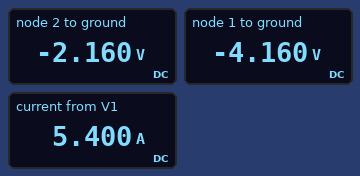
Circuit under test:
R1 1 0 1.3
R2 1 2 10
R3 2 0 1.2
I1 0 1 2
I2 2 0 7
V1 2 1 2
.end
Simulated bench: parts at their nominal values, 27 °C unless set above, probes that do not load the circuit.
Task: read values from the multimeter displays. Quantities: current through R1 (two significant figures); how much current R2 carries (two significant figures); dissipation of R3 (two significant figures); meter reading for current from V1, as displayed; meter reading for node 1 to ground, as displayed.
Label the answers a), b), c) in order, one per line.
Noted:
a) 3.2 A
b) 200 mA
c) 3.9 W
d) 5.400 A
e) -4.160 V
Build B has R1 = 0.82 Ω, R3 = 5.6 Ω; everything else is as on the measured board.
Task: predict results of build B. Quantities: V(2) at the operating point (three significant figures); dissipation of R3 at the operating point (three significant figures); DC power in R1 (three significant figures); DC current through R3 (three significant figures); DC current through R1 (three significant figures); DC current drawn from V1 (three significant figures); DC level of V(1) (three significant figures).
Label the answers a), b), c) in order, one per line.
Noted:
a) -1.83 V
b) 599 mW
c) 17.9 W
d) 327 mA
e) 4.67 A
f) 6.87 A
g) -3.83 V
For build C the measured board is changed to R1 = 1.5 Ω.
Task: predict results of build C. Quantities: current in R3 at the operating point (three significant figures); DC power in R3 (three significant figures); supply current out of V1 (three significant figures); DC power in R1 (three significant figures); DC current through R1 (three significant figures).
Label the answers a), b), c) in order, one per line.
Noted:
a) 2.04 A
b) 4.98 W
c) 5.16 A
d) 13.2 W
e) 2.96 A
